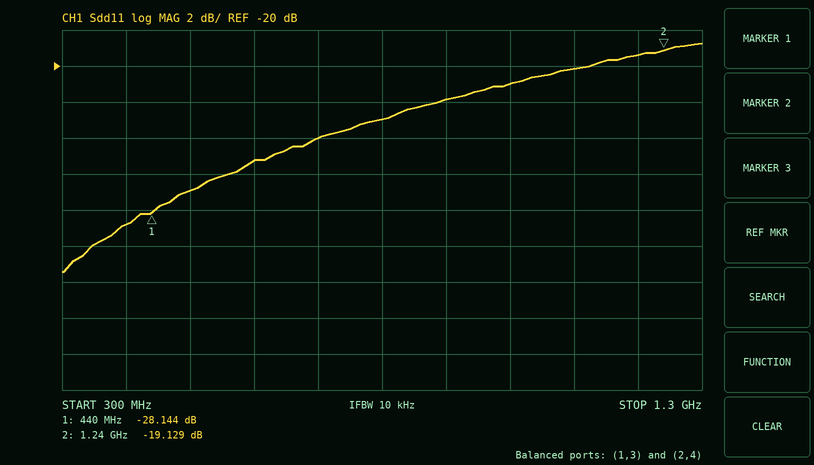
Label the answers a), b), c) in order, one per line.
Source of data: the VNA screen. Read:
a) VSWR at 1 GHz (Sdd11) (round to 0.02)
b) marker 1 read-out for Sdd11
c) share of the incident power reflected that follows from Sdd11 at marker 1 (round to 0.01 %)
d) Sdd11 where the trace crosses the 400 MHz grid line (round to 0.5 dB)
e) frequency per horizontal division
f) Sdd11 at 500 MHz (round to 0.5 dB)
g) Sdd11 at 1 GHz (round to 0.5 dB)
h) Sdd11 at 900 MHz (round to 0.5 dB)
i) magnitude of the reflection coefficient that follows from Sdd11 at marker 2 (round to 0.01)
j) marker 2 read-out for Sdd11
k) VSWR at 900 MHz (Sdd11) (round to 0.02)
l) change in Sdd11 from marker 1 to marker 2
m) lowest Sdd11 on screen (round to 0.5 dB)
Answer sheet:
a) 1.20
b) -28.144 dB
c) 0.15 %
d) -29.0 dB
e) 100 MHz
f) -27.0 dB
g) -21.0 dB
h) -22.0 dB
i) 0.11
j) -19.129 dB
k) 1.18
l) 9.015 dB
m) -31.5 dB
